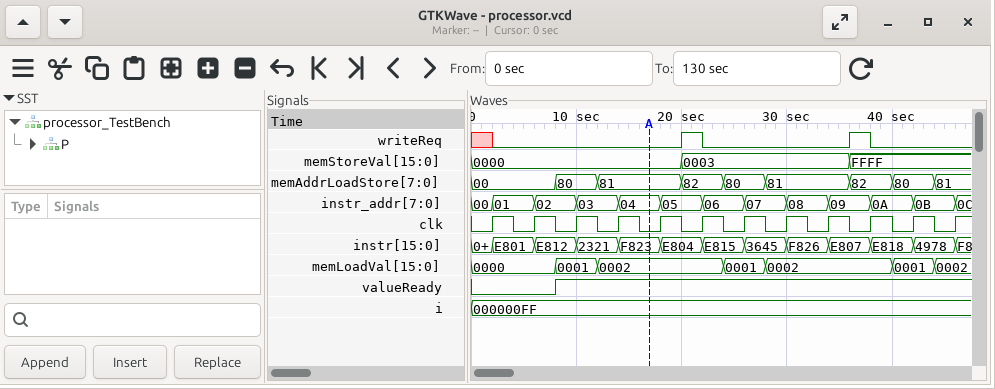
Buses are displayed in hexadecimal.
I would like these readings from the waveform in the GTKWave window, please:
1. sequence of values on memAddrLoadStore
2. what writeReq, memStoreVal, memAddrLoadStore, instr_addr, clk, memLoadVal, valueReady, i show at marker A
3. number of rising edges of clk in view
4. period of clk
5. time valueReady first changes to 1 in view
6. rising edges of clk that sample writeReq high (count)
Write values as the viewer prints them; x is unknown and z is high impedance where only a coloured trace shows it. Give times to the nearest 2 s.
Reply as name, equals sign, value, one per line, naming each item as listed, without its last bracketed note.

sequence of values on memAddrLoadStore = 00, 80, 81, 82, 80, 81, 82, 80, 81
what writeReq, memStoreVal, memAddrLoadStore, instr_addr, clk, memLoadVal, valueReady, i show at marker A = writeReq=0, memStoreVal=0000, memAddrLoadStore=81, instr_addr=04, clk=0, memLoadVal=0002, valueReady=1, i=000000FF
number of rising edges of clk in view = 12
period of clk = 4 s
time valueReady first changes to 1 in view = 8 s
rising edges of clk that sample writeReq high = 2
